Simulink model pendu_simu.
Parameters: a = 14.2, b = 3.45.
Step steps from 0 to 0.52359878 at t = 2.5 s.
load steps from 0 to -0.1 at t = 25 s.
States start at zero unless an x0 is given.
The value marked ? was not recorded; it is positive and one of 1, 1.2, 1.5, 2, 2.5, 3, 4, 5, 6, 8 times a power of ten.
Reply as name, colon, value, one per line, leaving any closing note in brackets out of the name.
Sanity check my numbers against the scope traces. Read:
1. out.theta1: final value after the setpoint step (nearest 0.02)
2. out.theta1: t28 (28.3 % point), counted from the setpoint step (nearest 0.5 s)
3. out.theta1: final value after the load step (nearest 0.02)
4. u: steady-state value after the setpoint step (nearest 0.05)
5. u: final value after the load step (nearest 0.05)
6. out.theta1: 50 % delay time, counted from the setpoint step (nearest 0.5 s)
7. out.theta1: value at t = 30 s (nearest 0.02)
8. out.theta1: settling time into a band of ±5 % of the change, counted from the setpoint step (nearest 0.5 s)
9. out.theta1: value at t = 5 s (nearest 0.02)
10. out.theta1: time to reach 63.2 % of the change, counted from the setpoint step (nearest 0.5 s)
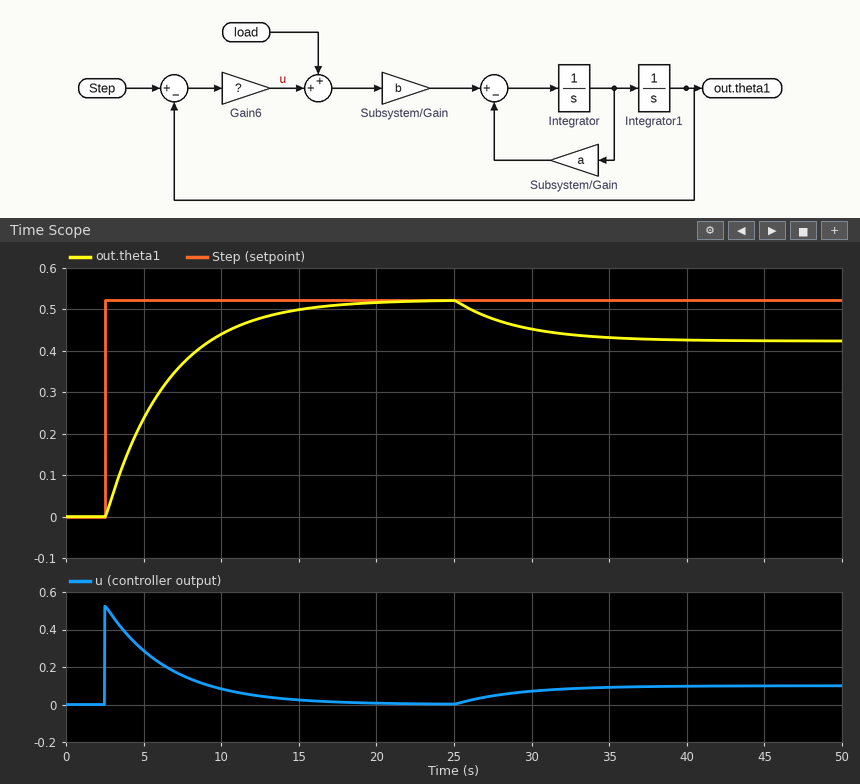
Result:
out.theta1: final value after the setpoint step: 0.52
out.theta1: t28 (28.3 % point), counted from the setpoint step: 1.5 s
out.theta1: final value after the load step: 0.42
u: steady-state value after the setpoint step: 0.00
u: final value after the load step: 0.10
out.theta1: 50 % delay time, counted from the setpoint step: 3.0 s
out.theta1: value at t = 30 s: 0.46
out.theta1: settling time into a band of ±5 % of the change, counted from the setpoint step: 12.0 s
out.theta1: value at t = 5 s: 0.24
out.theta1: time to reach 63.2 % of the change, counted from the setpoint step: 4.0 s
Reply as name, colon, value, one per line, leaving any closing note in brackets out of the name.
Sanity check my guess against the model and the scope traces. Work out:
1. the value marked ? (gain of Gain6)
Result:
the value marked ?: 1
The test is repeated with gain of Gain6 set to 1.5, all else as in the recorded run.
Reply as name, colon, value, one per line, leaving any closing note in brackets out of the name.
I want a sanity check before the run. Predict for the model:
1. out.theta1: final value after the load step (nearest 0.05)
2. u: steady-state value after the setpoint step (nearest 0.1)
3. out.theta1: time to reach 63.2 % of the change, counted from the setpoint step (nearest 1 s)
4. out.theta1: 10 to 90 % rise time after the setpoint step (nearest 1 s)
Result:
out.theta1: final value after the load step: 0.45
u: steady-state value after the setpoint step: 0.0
out.theta1: time to reach 63.2 % of the change, counted from the setpoint step: 3 s
out.theta1: 10 to 90 % rise time after the setpoint step: 6 s
